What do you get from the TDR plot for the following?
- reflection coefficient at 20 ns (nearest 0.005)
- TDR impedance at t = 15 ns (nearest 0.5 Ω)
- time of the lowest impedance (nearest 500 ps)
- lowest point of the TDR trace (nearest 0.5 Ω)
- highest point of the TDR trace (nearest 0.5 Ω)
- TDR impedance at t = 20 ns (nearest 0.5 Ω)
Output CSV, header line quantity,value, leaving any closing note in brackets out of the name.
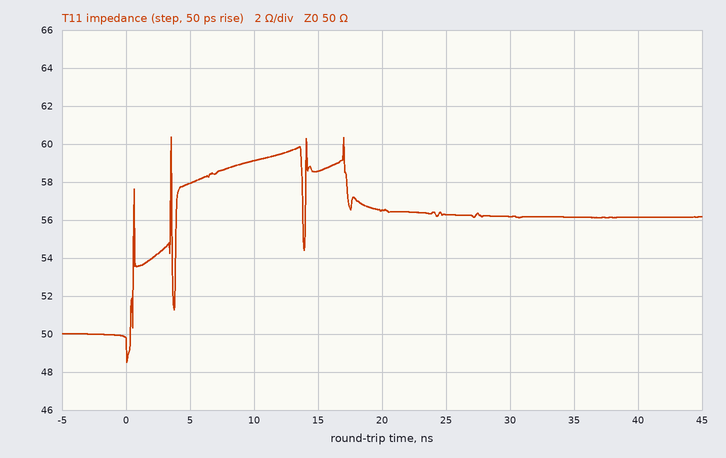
quantity,value
reflection coefficient at 20 ns,+0.060
TDR impedance at t = 15 ns,58.5 Ω
time of the lowest impedance,0.0 ns
lowest point of the TDR trace,48.5 Ω
highest point of the TDR trace,60.5 Ω
TDR impedance at t = 20 ns,56.5 Ω
